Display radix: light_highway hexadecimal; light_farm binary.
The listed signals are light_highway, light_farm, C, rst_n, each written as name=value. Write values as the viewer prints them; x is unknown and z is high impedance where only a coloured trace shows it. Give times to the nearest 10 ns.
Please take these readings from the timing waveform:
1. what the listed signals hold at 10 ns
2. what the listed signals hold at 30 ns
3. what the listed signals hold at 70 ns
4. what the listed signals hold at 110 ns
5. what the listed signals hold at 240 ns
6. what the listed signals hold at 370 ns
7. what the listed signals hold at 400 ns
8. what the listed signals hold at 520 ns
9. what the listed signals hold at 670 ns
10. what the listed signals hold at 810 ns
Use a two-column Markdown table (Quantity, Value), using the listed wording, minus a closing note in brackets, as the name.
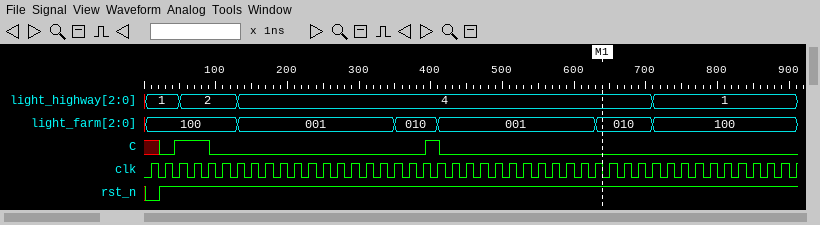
| Quantity | Value |
|---|---|
| what the listed signals hold at 10 ns | light_highway=1, light_farm=100, C=x, rst_n=0 |
| what the listed signals hold at 30 ns | light_highway=1, light_farm=100, C=0, rst_n=1 |
| what the listed signals hold at 70 ns | light_highway=2, light_farm=100, C=1, rst_n=1 |
| what the listed signals hold at 110 ns | light_highway=2, light_farm=100, C=0, rst_n=1 |
| what the listed signals hold at 240 ns | light_highway=4, light_farm=001, C=0, rst_n=1 |
| what the listed signals hold at 370 ns | light_highway=4, light_farm=010, C=0, rst_n=1 |
| what the listed signals hold at 400 ns | light_highway=4, light_farm=010, C=1, rst_n=1 |
| what the listed signals hold at 520 ns | light_highway=4, light_farm=001, C=0, rst_n=1 |
| what the listed signals hold at 670 ns | light_highway=4, light_farm=010, C=0, rst_n=1 |
| what the listed signals hold at 810 ns | light_highway=1, light_farm=100, C=0, rst_n=1 |
